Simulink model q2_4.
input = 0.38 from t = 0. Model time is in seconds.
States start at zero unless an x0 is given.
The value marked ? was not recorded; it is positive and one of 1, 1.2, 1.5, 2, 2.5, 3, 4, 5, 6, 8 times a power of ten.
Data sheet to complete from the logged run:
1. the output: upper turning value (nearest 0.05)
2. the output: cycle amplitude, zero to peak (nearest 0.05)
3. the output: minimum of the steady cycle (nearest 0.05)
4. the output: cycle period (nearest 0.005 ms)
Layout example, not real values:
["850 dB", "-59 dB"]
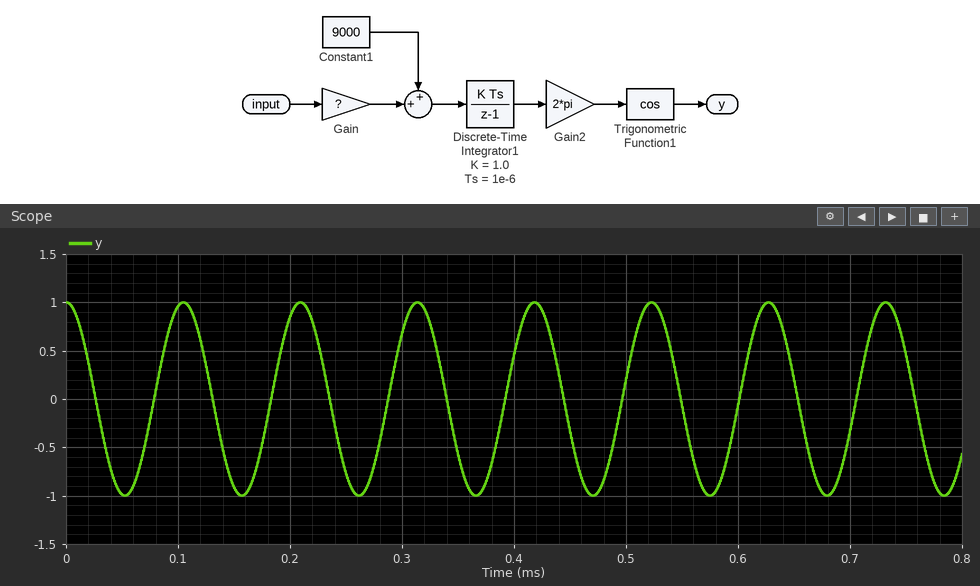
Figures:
["1.00", "1.00", "-1.00", "0.105 ms"]
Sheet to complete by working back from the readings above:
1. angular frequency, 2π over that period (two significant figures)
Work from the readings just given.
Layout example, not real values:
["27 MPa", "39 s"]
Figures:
["60 rad/ms"]
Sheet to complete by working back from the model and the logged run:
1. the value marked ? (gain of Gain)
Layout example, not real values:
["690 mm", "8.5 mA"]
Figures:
["1500"]
